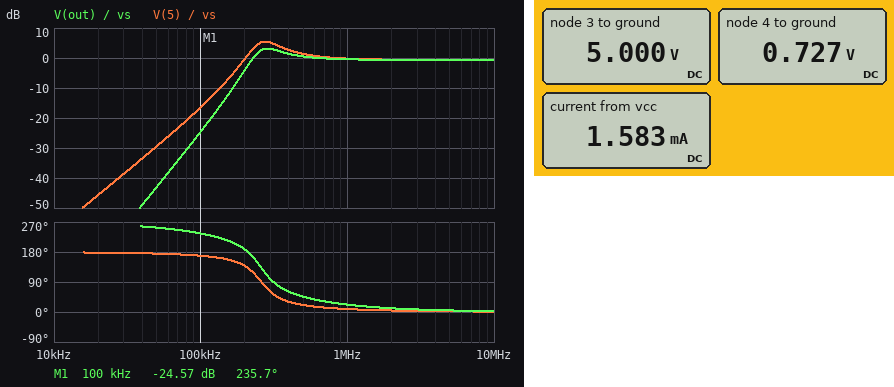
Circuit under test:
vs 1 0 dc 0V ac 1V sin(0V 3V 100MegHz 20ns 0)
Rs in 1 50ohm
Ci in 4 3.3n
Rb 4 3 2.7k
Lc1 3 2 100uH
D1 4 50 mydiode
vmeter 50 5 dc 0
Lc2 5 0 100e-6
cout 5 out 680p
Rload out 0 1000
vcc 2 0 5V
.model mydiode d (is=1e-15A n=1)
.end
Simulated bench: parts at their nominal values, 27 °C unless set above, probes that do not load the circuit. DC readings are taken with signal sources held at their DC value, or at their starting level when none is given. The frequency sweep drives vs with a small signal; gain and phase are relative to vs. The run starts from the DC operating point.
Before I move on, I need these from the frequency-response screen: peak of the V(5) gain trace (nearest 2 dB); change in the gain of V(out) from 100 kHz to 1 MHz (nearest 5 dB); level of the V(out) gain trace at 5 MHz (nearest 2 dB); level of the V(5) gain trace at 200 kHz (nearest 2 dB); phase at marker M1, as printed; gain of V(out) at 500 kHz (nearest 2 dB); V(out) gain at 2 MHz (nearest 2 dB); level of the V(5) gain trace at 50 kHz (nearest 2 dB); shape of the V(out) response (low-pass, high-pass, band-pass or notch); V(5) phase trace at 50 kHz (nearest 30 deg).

6 dB
25 dB
0 dB
0 dB
235.7 deg
0 dB
0 dB
-30 dB
high-pass
180 deg
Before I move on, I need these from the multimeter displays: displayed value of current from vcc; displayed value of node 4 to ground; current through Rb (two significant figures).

1.583 mA
0.727 V
1.6 mA
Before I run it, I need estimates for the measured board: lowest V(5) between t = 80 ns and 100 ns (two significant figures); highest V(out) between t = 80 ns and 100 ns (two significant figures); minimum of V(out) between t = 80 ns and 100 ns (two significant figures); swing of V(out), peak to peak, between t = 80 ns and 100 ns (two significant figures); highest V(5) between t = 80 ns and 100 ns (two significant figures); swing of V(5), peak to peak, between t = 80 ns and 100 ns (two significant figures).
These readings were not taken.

-1.8 V
2.8 V
-1.8 V
4.6 V
2.8 V
4.6 V
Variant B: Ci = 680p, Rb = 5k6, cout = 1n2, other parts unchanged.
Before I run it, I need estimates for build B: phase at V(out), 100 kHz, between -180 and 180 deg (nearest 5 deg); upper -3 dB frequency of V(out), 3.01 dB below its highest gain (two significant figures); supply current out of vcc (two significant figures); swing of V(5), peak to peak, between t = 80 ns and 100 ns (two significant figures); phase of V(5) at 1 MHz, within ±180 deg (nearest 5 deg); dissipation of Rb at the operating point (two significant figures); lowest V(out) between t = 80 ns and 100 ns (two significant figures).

-130 deg
1.3 MHz
770 µA
3.9 V
30 deg
3.3 mW
-1.2 V
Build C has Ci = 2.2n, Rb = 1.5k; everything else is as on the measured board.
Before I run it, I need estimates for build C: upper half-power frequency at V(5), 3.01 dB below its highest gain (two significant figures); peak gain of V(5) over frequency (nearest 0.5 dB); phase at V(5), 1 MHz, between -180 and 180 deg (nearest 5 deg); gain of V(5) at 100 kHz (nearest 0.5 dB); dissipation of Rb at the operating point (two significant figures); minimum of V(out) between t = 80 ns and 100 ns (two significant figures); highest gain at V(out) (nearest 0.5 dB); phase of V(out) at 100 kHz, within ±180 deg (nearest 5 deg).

530 kHz
5.0 dB
10 deg
-20.5 dB
12 mW
-2.8 V
3.5 dB
-120 deg
